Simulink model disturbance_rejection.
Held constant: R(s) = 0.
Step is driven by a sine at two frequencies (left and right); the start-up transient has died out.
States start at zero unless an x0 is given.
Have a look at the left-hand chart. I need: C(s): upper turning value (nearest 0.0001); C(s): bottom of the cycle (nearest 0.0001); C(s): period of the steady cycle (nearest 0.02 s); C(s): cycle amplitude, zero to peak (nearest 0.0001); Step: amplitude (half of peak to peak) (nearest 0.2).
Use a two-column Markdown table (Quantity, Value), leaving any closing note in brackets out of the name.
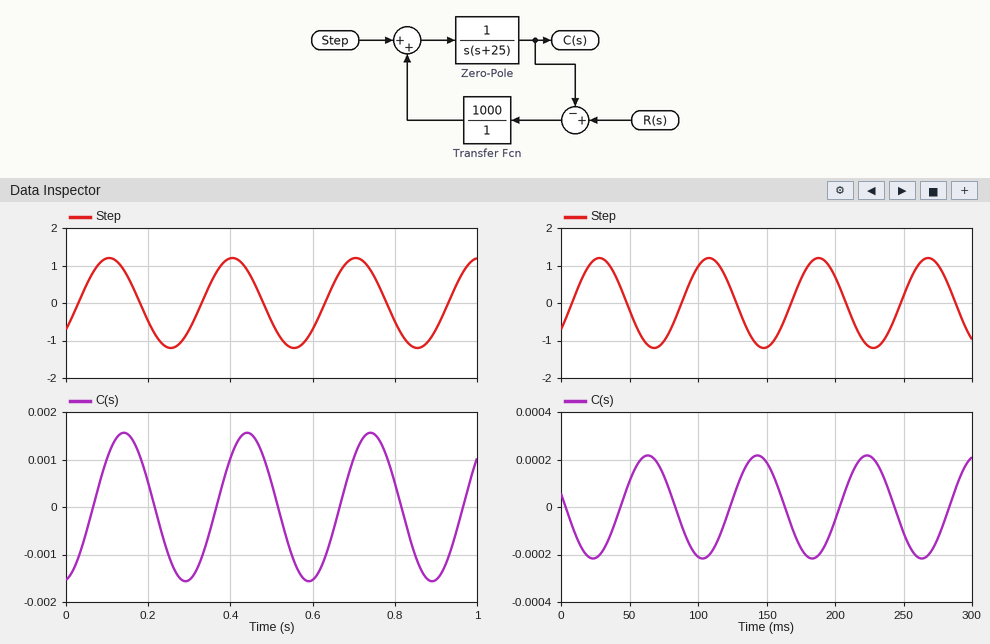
| Quantity | Value |
|---|---|
| C(s): upper turning value | 0.0016 |
| C(s): bottom of the cycle | -0.0016 |
| C(s): period of the steady cycle | 0.30 s |
| C(s): cycle amplitude, zero to peak | 0.0016 |
| Step: amplitude (half of peak to peak) | 1.2 |
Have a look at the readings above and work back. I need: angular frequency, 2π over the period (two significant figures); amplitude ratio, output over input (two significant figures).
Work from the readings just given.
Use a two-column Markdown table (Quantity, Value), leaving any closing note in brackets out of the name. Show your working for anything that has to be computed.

| Quantity | Value |
|---|---|
| angular frequency, 2π over the period | 2π / 0.3 = 21 rad/s |
| amplitude ratio, output over input | 0.0016 / 1.2 = 0.0013 |
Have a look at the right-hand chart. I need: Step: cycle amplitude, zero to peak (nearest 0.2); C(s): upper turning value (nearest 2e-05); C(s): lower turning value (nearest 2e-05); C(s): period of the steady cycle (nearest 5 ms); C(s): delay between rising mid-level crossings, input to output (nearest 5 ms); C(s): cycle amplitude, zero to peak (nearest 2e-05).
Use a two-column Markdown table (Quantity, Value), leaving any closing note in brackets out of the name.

| Quantity | Value |
|---|---|
| Step: cycle amplitude, zero to peak | 1.2 |
| C(s): upper turning value | 0.00022 |
| C(s): lower turning value | -0.00022 |
| C(s): period of the steady cycle | 80 ms |
| C(s): delay between rising mid-level crossings, input to output | 35 ms |
| C(s): cycle amplitude, zero to peak | 0.00022 |
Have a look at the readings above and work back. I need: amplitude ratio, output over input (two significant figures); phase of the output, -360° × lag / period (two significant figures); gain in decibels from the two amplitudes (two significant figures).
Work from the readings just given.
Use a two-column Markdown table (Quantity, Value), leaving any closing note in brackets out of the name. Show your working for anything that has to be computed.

| Quantity | Value |
|---|---|
| amplitude ratio, output over input | 0.00022 / 1.2 = 0.00018 |
| phase of the output, -360° × lag / period | -360 × 35 / 80 = -160° |
| gain in decibels from the two amplitudes | 20 log10(0.00022 / 1.2) = -75 dB |
